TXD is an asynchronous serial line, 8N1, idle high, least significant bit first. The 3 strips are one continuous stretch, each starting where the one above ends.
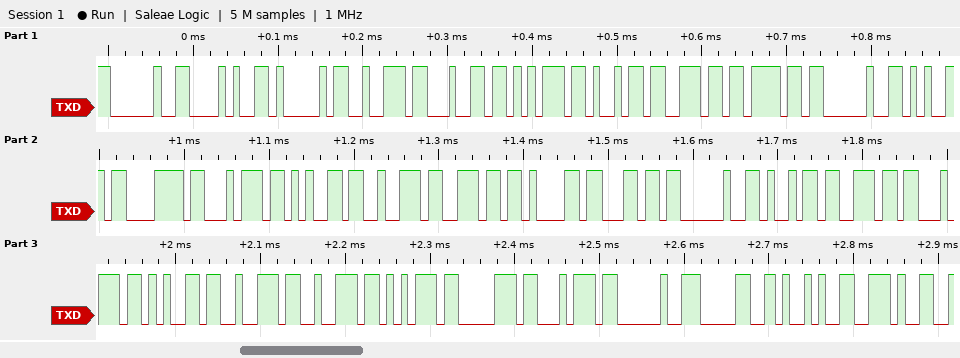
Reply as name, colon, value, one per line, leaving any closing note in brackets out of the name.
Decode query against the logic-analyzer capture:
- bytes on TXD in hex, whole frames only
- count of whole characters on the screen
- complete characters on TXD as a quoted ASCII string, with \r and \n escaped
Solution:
bytes on TXD in hex, whole frames only: 0x20 0x28 0x41 0x72 0x64 0x75 0x69 0x6E 0x6F 0x20 0x65 0x78 0x74 0x65 0x72 0x6E 0x61 0x6C 0x20 0x69 0x6E 0x74 0x65 0x72 0x72 0x75 0x70 0x74 0x20 0x30 0x29 0x2E
count of whole characters on the screen: 32
complete characters on TXD as a quoted ASCII string, with \r and \n escaped: " (Arduino external interrupt 0)."
